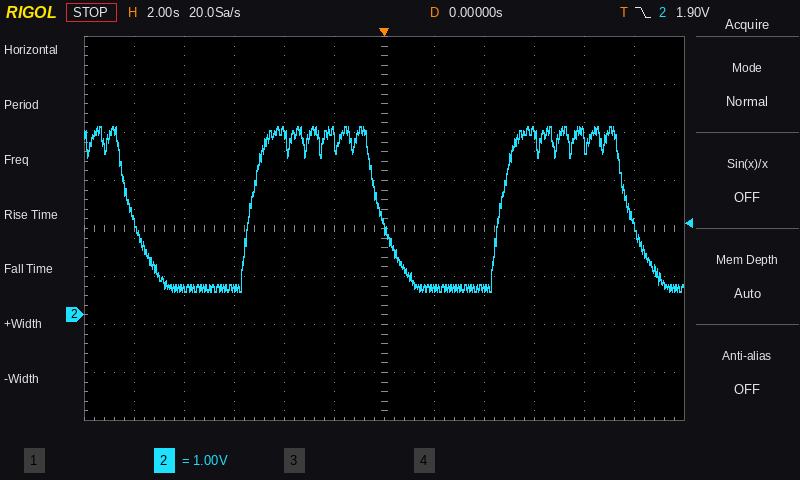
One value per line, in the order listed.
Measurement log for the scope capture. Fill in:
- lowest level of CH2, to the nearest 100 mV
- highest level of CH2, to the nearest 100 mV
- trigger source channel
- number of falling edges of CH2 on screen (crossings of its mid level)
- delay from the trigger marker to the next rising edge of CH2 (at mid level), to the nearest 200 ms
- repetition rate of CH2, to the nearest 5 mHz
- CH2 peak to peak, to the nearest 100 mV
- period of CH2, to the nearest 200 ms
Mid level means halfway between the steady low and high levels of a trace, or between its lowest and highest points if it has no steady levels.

500 mV
3.9 V
CH2
3
4.6 s
100 mHz
3.4 V
10.0 s
